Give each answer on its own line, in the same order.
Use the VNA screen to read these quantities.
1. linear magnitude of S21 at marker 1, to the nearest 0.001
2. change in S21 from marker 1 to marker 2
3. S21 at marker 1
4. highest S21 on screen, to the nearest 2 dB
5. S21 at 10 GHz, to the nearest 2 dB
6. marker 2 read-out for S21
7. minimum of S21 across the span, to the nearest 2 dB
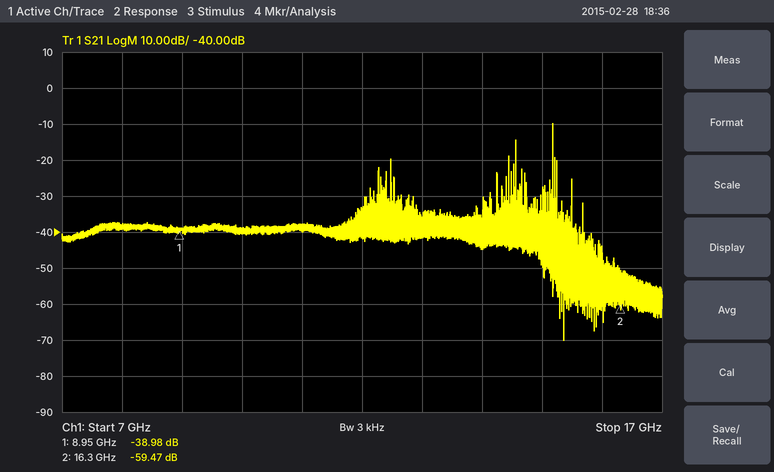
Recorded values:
0.011
-20.49 dB
-38.98 dB
-10 dB
-40 dB
-59.47 dB
-70 dB
